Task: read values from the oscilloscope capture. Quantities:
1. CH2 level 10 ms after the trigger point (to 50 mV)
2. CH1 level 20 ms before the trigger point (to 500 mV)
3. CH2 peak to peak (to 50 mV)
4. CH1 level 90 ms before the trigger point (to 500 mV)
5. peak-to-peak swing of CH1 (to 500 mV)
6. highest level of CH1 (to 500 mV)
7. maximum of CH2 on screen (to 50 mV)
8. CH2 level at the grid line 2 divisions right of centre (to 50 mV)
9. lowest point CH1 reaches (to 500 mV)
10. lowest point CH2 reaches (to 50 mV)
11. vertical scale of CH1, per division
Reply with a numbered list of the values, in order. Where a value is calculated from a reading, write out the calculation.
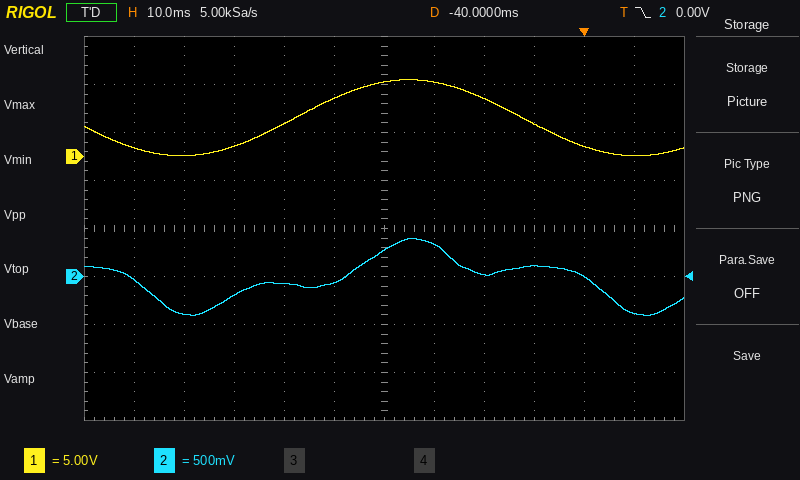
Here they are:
1. -400 mV
2. 6.0 V
3. 400 mV − (-400 mV) = 800 mV
4. 1.0 V
5. 8.0 V − (0.0 V) = 8.0 V
6. 8.0 V
7. 400 mV
8. 0 mV
9. 0.0 V
10. -400 mV
11. 5 V
